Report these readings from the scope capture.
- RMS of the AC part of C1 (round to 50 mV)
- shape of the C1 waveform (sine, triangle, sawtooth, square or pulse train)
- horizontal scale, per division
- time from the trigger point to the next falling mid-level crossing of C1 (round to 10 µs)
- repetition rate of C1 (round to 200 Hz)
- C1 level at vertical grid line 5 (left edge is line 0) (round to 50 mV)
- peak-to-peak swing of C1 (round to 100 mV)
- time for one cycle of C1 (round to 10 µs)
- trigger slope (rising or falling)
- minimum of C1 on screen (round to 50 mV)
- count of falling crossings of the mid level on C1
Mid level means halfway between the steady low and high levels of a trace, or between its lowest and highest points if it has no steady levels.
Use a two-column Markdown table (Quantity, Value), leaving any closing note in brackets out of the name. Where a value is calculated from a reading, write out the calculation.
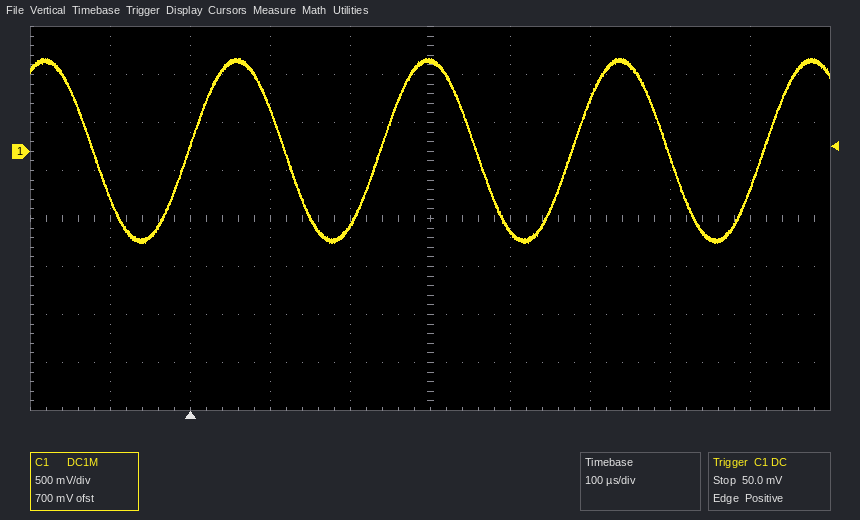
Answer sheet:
| Quantity | Value |
|---|---|
| RMS of the AC part of C1 | 1.90 V / (2√2) ≈ 672 mV, so 650 mV to the nearest 50 mV |
| shape of the C1 waveform | sine |
| horizontal scale, per division | 100 µs |
| time from the trigger point to the next falling mid-level crossing of C1 | 120 µs |
| repetition rate of C1 | 1 / 240 µs ≈ 4.2 kHz |
| C1 level at vertical grid line 5 (left edge is line 0) | 950 mV |
| peak-to-peak swing of C1 | 1.90 V |
| time for one cycle of C1 | 240 µs |
| trigger slope | rising |
| minimum of C1 on screen | -950 mV |
| count of falling crossings of the mid level on C1 | 4 |
